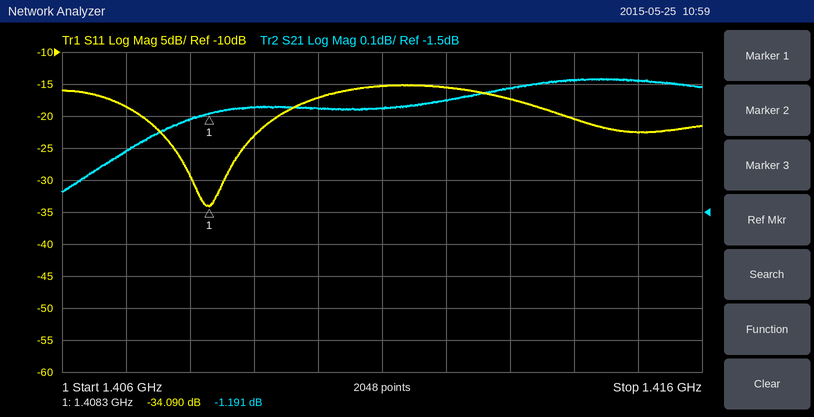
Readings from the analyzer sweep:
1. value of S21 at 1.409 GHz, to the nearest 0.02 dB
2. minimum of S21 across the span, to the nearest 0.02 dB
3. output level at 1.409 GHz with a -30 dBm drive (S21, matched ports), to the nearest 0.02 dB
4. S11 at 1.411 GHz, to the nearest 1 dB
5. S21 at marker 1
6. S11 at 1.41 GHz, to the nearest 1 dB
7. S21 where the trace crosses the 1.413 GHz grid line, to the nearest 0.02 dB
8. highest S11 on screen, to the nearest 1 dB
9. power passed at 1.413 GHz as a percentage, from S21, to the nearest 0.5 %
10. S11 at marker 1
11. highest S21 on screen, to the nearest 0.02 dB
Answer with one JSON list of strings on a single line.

["-1.18 dB", "-1.44 dB", "-31.18 dBm", "-15 dB", "-1.191 dB", "-17 dB", "-1.12 dB", "-15 dB", "77.5 %", "-34.090 dB", "-1.08 dB"]
